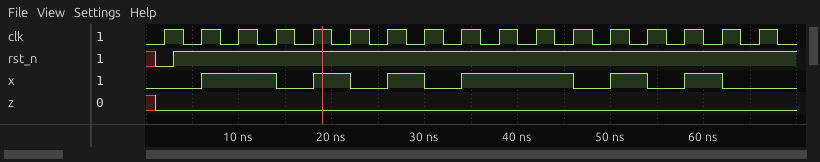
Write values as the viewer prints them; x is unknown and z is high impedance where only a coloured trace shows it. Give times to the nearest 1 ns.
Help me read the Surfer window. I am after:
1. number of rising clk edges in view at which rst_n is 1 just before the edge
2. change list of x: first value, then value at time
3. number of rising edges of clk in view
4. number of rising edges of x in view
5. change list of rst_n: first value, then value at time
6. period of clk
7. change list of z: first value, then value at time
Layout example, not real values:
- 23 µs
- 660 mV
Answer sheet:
- 16
- 0, 1 at 6 ns, 0 at 14 ns, 1 at 18 ns, 0 at 22 ns, 1 at 26 ns, 0 at 30 ns, 1 at 34 ns, 0 at 46 ns, 1 at 50 ns, 0 at 54 ns, 1 at 58 ns, 0 at 62 ns
- 17
- 6
- x, 0 at 1 ns, 1 at 3 ns
- 4 ns
- x, 0 at 1 ns
